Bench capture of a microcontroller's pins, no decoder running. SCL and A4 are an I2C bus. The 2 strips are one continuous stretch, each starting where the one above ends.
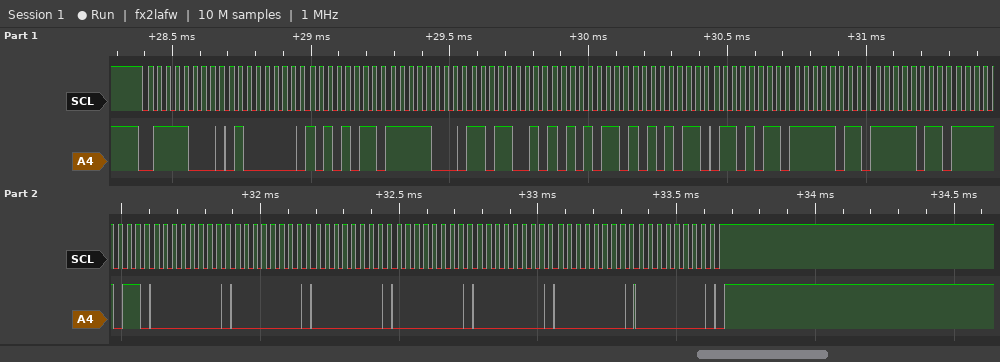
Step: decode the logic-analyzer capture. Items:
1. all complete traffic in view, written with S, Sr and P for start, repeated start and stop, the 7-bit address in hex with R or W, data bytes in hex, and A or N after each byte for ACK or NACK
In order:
S 3CW A 40 A AB A F8 A D9 A AB A AB A 6B A FB A FB A FB A 00 A 00 A 00 A 00 A 00 A 00 A 00 A P
